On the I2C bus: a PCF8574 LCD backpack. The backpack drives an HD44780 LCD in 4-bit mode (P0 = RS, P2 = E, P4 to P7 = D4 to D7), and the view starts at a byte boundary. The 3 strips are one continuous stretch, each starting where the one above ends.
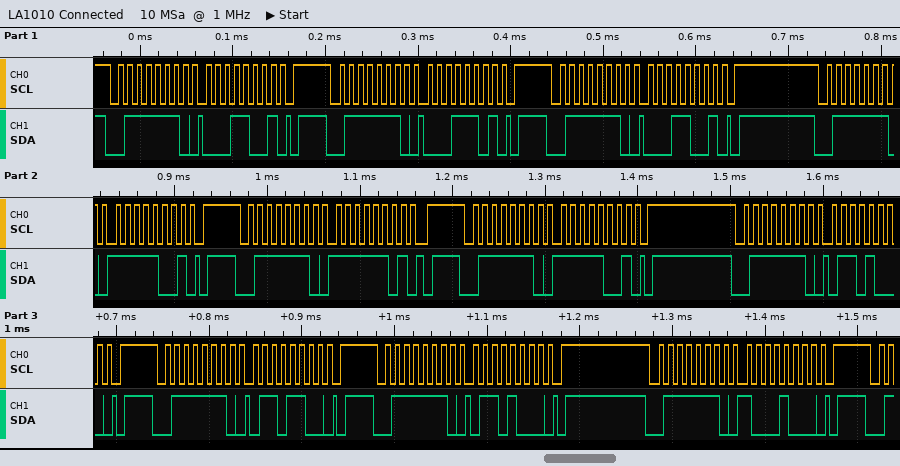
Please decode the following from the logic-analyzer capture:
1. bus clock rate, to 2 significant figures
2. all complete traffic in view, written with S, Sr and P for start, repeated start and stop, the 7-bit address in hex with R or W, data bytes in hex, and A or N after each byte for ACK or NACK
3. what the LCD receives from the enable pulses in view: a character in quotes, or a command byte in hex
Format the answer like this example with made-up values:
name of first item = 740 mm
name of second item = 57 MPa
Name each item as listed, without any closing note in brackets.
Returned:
bus clock rate, to 2 significant figures = 100 kHz
all complete traffic in view, written with S, Sr and P for start, repeated start and stop, the 7-bit address in hex with R or W, data bytes in hex, and A or N after each byte for ACK or NACK = S 3FW A 19 A P S 3FW A 1D A P S 3FW A 19 A P S 3FW A F9 A P S 3FW A FD A P S 3FW A F9 A P S 3FW A 68 A P S 3FW A 6C A P S 3FW A 68 A P S 3FW A 88 A P
what the LCD receives from the enable pulses in view: a character in quotes, or a command byte in hex = data 0x1F
